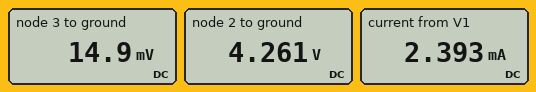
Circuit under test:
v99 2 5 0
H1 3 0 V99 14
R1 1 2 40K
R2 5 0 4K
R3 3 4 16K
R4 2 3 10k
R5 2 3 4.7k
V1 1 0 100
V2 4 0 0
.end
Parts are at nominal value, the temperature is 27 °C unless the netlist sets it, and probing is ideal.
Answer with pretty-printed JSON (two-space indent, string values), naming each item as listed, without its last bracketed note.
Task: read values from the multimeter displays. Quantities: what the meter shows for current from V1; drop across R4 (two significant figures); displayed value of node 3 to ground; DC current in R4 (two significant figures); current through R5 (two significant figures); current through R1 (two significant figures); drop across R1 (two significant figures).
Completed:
{
  "what the meter shows for current from V1": "2.393 mA",
  "drop across R4": "4.2 V",
  "displayed value of node 3 to ground": "14.9 mV",
  "DC current in R4": "420 µA",
  "current through R5": "900 µA",
  "current through R1": "2.4 mA",
  "drop across R1": "96 V"
}
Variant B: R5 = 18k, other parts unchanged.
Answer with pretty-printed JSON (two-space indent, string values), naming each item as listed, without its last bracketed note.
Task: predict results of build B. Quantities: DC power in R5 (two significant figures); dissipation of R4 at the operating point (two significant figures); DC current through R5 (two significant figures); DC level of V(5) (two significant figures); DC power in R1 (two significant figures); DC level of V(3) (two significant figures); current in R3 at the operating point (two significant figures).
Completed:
{
  "DC power in R5": "1.9 mW",
  "dissipation of R4 at the operating point": "3.4 mW",
  "DC current through R5": "320 µA",
  "DC level of V(5)": "5.8 V",
  "DC power in R1": "220 mW",
  "DC level of V(3)": "20 mV",
  "current in R3 at the operating point": "1.3 µA"
}
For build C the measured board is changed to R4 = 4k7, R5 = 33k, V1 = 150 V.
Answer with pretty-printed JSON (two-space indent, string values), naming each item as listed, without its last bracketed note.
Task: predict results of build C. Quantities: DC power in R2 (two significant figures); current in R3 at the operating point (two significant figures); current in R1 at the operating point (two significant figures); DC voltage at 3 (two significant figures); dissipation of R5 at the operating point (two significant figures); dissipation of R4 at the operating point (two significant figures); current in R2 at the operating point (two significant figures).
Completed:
{
  "DC power in R2": "13 mW",
  "current in R3 at the operating point": "1.6 µA",
  "current in R1 at the operating point": "3.6 mA",
  "DC voltage at 3": "25 mV",
  "dissipation of R5 at the operating point": "1.6 mW",
  "dissipation of R4 at the operating point": "11 mW",
  "current in R2 at the operating point": "1.8 mA"
}
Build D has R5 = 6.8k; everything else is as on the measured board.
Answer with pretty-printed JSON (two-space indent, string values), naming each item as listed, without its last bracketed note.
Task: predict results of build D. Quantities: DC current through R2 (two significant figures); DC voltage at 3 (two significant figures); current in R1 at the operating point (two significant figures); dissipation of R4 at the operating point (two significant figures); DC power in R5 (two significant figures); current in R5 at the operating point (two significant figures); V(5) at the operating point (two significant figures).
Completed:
{
  "DC current through R2": "1.2 mA",
  "DC voltage at 3": "17 mV",
  "current in R1 at the operating point": "2.4 mA",
  "dissipation of R4 at the operating point": "2.3 mW",
  "DC power in R5": "3.4 mW",
  "current in R5 at the operating point": "700 µA",
  "V(5) at the operating point": "4.8 V"
}
